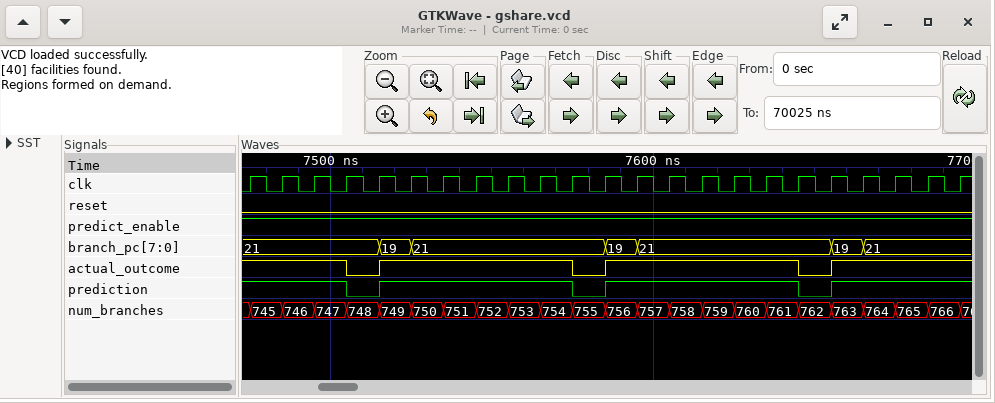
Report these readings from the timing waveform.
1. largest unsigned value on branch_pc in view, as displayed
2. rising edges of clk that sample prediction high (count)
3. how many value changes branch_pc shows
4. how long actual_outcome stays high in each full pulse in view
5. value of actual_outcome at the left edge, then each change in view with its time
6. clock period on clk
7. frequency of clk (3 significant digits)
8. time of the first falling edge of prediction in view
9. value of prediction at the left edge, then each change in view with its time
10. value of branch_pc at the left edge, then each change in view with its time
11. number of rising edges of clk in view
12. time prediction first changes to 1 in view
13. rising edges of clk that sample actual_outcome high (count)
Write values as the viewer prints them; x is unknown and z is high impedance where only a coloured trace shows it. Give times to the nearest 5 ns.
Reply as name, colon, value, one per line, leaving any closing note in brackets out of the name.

largest unsigned value on branch_pc in view, as displayed: 21
rising edges of clk that sample prediction high: 20
how many value changes branch_pc shows: 6
how long actual_outcome stays high in each full pulse in view: 60 ns, 60 ns
value of actual_outcome at the left edge, then each change in view with its time: 1, 0 at 7505 ns, 1 at 7515 ns, 0 at 7575 ns, 1 at 7585 ns, 0 at 7645 ns, 1 at 7655 ns
clock period on clk: 10 ns
frequency of clk: 100 MHz
time of the first falling edge of prediction in view: 7505 ns
value of prediction at the left edge, then each change in view with its time: 1, 0 at 7505 ns, 1 at 7515 ns, 0 at 7575 ns, 1 at 7585 ns, 0 at 7645 ns, 1 at 7655 ns
value of branch_pc at the left edge, then each change in view with its time: 21, 19 at 7515 ns, 21 at 7525 ns, 19 at 7585 ns, 21 at 7595 ns, 19 at 7655 ns, 21 at 7665 ns
number of rising edges of clk in view: 23
time prediction first changes to 1 in view: 7515 ns
rising edges of clk that sample actual_outcome high: 20
